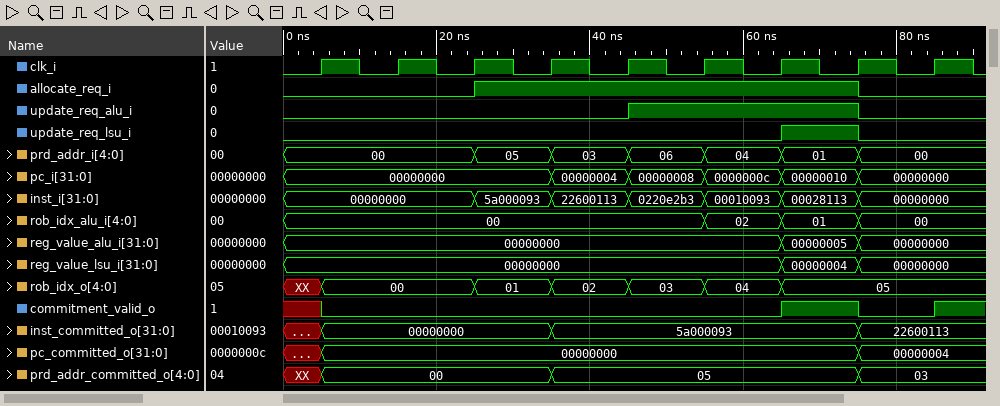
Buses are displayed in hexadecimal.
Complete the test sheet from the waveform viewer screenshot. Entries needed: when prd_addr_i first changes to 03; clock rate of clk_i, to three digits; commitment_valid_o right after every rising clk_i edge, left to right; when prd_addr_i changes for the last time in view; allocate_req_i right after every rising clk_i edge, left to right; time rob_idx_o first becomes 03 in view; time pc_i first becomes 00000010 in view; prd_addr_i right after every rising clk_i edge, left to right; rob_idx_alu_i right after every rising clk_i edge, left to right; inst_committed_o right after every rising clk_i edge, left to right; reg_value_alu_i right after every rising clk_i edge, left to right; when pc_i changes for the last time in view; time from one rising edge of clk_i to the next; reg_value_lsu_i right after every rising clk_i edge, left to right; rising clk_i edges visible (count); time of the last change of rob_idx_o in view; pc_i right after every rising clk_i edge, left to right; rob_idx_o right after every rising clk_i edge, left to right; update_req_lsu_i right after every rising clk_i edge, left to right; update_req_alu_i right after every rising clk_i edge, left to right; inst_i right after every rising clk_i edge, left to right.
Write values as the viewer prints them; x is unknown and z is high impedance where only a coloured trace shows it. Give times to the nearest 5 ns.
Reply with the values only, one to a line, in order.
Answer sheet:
35 ns
100 MHz
0 0 0 0 0 0 1 0 1
75 ns
0 0 1 1 1 1 1 0 0
45 ns
65 ns
00, 00, 05, 03, 06, 04, 01, 00, 00
00, 00, 00, 00, 00, 02, 01, 00, 00
00000000, 00000000, 00000000, 5a000093, 5a000093, 5a000093, 5a000093, 22600113, 22600113
00000000, 00000000, 00000000, 00000000, 00000000, 00000000, 00000005, 00000000, 00000000
75 ns
10 ns
00000000, 00000000, 00000000, 00000000, 00000000, 00000000, 00000004, 00000000, 00000000
9
65 ns
00000000, 00000000, 00000000, 00000004, 00000008, 0000000c, 00000010, 00000000, 00000000
00, 00, 01, 02, 03, 04, 05, 05, 05
0 0 0 0 0 0 1 0 0
0 0 0 0 1 1 1 0 0
00000000, 00000000, 5a000093, 22600113, 0220e2b3, 00010093, 00028113, 00000000, 00000000
